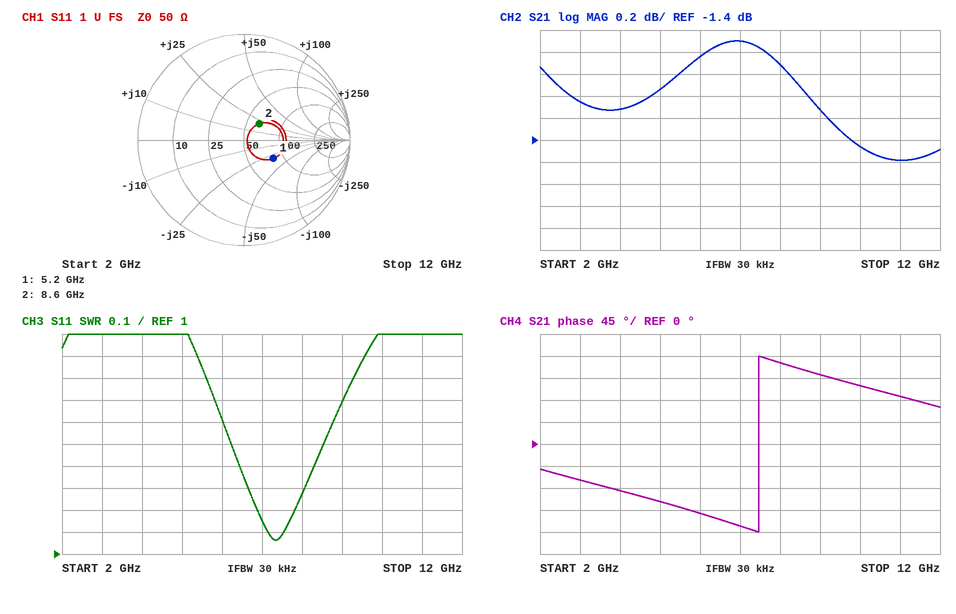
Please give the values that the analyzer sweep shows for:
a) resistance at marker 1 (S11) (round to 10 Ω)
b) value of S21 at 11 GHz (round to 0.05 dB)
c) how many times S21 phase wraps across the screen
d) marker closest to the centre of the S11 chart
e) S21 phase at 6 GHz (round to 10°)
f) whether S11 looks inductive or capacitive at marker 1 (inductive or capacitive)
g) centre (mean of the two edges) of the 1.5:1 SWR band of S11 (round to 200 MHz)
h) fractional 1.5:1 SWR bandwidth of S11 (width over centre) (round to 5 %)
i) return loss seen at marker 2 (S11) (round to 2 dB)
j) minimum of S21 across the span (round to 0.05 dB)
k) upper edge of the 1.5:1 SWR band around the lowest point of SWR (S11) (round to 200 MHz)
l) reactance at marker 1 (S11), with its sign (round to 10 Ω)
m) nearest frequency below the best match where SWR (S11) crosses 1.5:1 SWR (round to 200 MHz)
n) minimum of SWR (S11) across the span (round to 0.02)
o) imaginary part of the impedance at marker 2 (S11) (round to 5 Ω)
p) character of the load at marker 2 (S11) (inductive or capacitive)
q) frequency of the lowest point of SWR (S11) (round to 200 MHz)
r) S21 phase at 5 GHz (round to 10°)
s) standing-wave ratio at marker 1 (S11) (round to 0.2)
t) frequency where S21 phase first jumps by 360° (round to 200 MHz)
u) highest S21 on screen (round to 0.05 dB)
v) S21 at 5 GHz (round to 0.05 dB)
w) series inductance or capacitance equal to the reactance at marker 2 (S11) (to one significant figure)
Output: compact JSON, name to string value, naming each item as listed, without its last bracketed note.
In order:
{"resistance at marker 1 (S11)": "80 Ω", "value of S21 at 11 GHz": "-1.60 dB", "how many times S21 phase wraps across the screen": "1", "marker closest to the centre of the S11 chart": "marker 2", "S21 phase at 6 GHz": "-140°", "whether S11 looks inductive or capacitive at marker 1": "capacitive", "centre (mean of the two edges) of the 1.5:1 SWR band of S11": "7.4 GHz", "fractional 1.5:1 SWR bandwidth of S11 (width over centre)": "30 %", "return loss seen at marker 2 (S11)": "14 dB", "minimum of S21 across the span": "-1.60 dB", "upper edge of the 1.5:1 SWR band around the lowest point of SWR (S11)": "8.6 GHz", "reactance at marker 1 (S11), with its sign": "-30 Ω", "nearest frequency below the best match where SWR (S11) crosses 1.5:1 SWR": "6.2 GHz", "minimum of SWR (S11) across the span": "1.06", "imaginary part of the impedance at marker 2 (S11)": "+20 Ω", "character of the load at marker 2 (S11)": "inductive", "frequency of the lowest point of SWR (S11)": "7.4 GHz", "S21 phase at 5 GHz": "-120°", "standing-wave ratio at marker 1 (S11)": "2.0", "frequency where S21 phase first jumps by 360°": "7.4 GHz", "highest S21 on screen": "-0.50 dB", "S21 at 5 GHz": "-0.95 dB", "series inductance or capacitance equal to the reactance at marker 2 (S11)": "400 pH"}
